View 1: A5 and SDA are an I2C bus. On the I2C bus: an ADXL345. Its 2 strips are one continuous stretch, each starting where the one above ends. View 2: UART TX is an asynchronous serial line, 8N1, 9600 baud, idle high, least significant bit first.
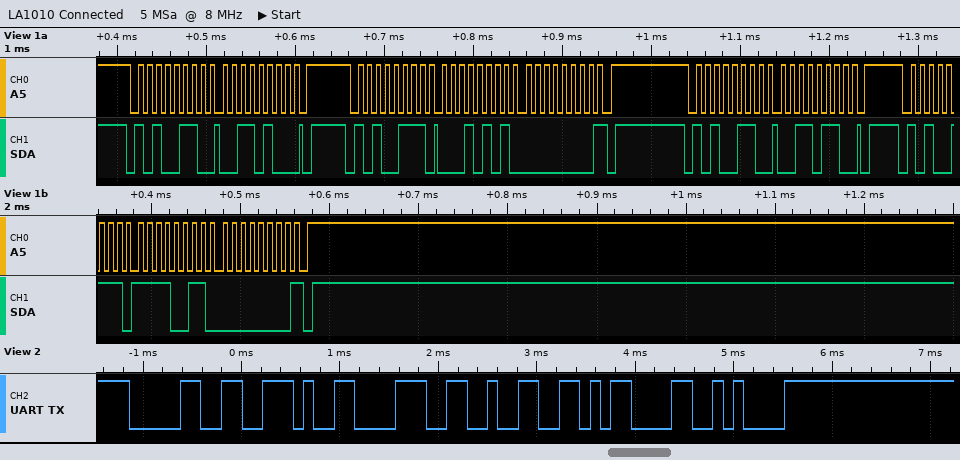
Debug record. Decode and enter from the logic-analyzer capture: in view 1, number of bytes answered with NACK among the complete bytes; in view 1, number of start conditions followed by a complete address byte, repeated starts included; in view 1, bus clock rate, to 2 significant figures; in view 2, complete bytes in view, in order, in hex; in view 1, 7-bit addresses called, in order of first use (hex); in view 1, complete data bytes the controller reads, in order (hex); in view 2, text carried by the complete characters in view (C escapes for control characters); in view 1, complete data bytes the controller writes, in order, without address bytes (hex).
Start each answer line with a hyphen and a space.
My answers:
- 2
- 4
- 100 kHz
- 0x30 0x2E 0x38 0x32 0x0D 0x0A
- 0x53
- 15 00 F3 00
- "0.82\r\n"
- 34 36
